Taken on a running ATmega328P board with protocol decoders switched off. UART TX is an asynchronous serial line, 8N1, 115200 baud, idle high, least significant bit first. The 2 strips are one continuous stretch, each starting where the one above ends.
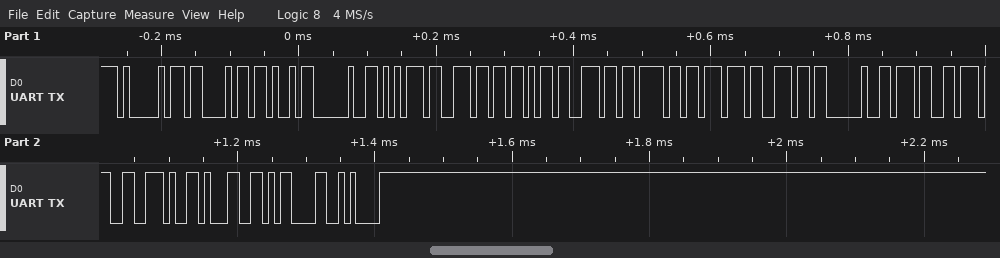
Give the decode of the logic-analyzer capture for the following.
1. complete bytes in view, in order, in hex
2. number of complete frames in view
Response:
0x41 0x43 0x4B 0x20 0x75 0x6E 0x6B 0x6E 0x6F 0x77 0x6E 0x20 0x37 0x37 0x2E 0x31 0x0D 0x0A
18
